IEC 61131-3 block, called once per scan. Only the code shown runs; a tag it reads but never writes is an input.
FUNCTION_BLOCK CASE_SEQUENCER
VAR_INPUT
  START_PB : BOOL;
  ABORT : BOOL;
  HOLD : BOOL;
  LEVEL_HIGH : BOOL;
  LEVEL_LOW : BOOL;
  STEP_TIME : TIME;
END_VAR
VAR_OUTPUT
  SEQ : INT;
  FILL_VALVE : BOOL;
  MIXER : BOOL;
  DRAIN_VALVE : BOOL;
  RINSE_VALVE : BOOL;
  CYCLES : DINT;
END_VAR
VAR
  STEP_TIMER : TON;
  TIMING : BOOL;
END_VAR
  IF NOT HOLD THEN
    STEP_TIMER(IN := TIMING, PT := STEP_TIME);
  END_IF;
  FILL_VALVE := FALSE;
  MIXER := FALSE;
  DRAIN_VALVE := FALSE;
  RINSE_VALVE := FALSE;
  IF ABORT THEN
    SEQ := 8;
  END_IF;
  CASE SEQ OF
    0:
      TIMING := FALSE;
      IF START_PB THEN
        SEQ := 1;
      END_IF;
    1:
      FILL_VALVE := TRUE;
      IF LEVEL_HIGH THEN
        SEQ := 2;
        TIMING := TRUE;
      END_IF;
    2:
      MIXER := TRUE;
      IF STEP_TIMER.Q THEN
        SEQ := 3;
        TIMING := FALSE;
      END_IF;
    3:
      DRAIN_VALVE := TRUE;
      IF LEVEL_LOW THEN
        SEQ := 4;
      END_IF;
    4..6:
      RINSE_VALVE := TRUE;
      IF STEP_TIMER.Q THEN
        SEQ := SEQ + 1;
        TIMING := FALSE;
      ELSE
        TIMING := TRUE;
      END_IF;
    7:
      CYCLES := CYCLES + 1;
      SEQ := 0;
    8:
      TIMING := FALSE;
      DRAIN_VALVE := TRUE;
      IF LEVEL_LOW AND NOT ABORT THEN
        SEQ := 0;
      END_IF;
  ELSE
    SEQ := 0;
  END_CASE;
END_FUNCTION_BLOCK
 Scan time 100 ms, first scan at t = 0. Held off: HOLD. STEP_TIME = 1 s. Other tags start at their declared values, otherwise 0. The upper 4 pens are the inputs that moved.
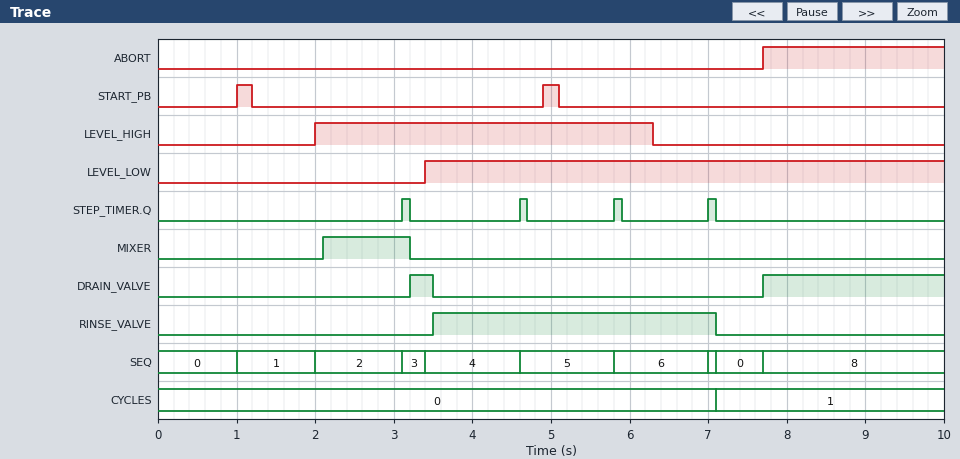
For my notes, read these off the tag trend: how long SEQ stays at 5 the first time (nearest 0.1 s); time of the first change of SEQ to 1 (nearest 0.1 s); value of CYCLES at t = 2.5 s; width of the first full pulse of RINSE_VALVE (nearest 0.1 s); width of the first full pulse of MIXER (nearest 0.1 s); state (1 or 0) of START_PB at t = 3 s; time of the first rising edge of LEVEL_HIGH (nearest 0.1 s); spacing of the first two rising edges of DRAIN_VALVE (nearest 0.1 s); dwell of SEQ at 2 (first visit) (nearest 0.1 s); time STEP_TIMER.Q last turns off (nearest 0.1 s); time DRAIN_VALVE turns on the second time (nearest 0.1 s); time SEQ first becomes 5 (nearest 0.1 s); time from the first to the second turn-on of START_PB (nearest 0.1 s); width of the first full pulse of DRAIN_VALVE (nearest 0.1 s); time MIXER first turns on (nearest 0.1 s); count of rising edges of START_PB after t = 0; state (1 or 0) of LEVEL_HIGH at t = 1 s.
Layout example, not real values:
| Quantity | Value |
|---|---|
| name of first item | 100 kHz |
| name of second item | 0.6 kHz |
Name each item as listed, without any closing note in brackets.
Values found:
| Quantity | Value |
|---|---|
| how long SEQ stays at 5 the first time | 1.2 s |
| time of the first change of SEQ to 1 | 1.0 s |
| value of CYCLES at t = 2.5 s | 0 |
| width of the first full pulse of RINSE_VALVE | 3.6 s |
| width of the first full pulse of MIXER | 1.1 s |
| state (1 or 0) of START_PB at t = 3 s | 0 |
| time of the first rising edge of LEVEL_HIGH | 2.0 s |
| spacing of the first two rising edges of DRAIN_VALVE | 4.5 s |
| dwell of SEQ at 2 (first visit) | 1.1 s |
| time STEP_TIMER.Q last turns off | 7.1 s |
| time DRAIN_VALVE turns on the second time | 7.7 s |
| time SEQ first becomes 5 | 4.6 s |
| time from the first to the second turn-on of START_PB | 3.9 s |
| width of the first full pulse of DRAIN_VALVE | 0.3 s |
| time MIXER first turns on | 2.1 s |
| count of rising edges of START_PB after t = 0 | 2 |
| state (1 or 0) of LEVEL_HIGH at t = 1 s | 0 |
